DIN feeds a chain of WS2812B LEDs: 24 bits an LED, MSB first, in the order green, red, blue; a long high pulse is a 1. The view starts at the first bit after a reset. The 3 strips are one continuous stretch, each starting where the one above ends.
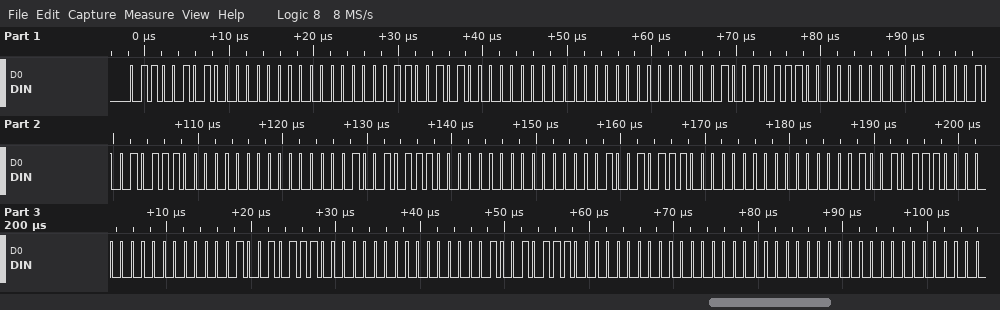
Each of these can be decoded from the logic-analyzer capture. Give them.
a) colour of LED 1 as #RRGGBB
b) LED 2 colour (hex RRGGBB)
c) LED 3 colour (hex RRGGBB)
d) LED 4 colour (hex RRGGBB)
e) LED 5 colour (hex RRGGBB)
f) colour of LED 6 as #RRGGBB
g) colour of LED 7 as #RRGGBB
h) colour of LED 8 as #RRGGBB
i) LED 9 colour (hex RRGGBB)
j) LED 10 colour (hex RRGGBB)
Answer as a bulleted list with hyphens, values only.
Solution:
- #006500
- #006500
- #970000
- #970000
- #970000
- #970000
- #970000
- #970000
- #970000
- #000000
